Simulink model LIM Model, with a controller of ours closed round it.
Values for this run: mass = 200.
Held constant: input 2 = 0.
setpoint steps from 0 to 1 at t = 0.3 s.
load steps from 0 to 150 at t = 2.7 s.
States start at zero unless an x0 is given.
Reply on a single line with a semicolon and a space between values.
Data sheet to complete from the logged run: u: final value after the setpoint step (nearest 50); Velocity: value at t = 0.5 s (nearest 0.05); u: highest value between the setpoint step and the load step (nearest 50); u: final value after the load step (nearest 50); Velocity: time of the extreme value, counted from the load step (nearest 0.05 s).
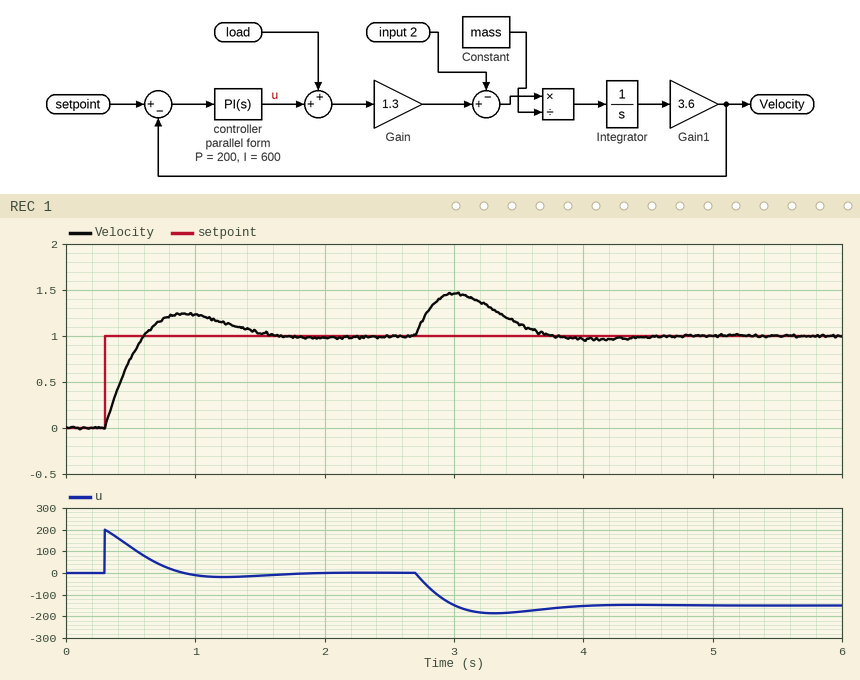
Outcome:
0; 0.75; 200; -150; 0.30 s
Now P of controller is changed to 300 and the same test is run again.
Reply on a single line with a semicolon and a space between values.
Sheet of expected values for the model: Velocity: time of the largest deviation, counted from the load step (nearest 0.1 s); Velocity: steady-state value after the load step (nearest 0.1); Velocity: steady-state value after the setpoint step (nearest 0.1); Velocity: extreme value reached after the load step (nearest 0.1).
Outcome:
0.3 s; 1.0; 1.0; 1.4
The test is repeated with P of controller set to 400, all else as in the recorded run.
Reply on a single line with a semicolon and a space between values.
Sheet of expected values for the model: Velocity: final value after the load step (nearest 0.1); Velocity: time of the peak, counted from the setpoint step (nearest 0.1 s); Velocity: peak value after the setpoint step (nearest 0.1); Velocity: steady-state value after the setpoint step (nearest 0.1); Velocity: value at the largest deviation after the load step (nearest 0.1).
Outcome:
1.0; 0.5 s; 1.1; 1.0; 1.3
